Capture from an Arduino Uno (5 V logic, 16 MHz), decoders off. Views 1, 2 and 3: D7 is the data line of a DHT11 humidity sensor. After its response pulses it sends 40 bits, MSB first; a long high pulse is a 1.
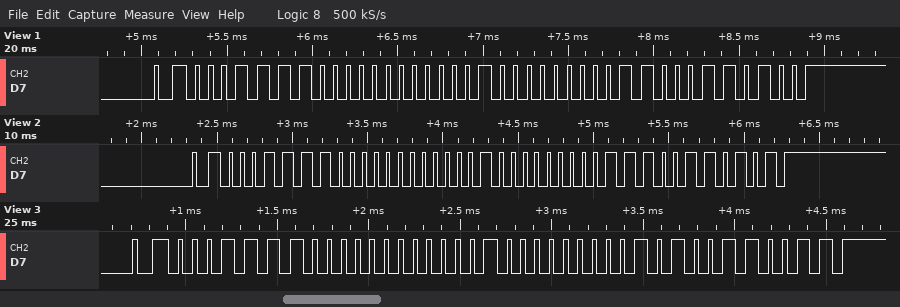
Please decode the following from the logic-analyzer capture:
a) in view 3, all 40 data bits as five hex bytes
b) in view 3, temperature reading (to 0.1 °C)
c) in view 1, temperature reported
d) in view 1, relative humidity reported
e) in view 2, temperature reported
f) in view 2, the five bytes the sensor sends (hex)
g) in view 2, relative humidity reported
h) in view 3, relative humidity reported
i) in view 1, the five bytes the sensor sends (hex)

1E 00 10 05 33
16.5 °C
16.6 °C
30 %
16.7 °C
1E 00 10 07 35
30 %
30 %
1E 00 10 06 34
